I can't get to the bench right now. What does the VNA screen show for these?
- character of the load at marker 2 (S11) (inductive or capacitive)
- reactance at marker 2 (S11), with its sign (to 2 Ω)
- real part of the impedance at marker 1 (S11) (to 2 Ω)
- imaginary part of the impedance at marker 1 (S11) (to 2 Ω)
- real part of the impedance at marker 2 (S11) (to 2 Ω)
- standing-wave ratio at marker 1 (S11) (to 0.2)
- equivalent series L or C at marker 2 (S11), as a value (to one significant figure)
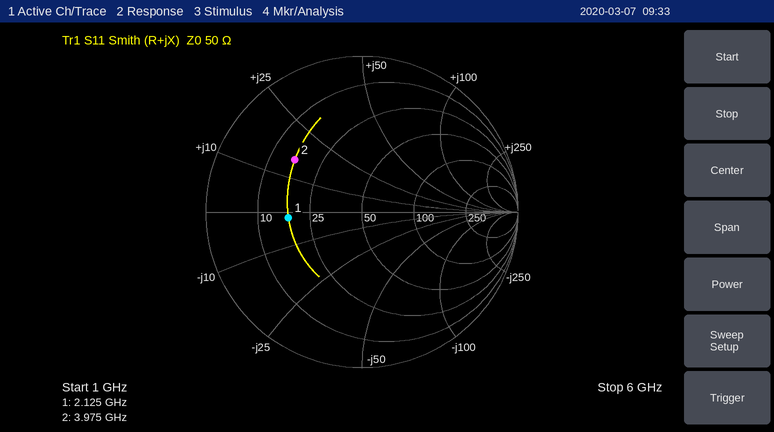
inductive
+16 Ω
18 Ω
-2 Ω
16 Ω
2.8
600 pH
